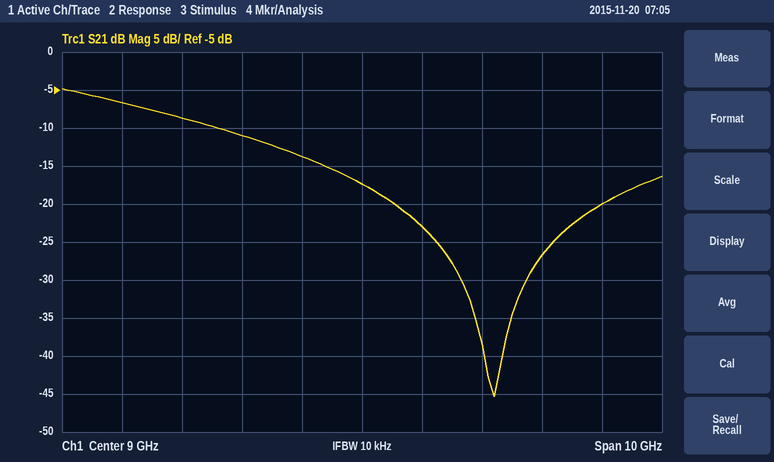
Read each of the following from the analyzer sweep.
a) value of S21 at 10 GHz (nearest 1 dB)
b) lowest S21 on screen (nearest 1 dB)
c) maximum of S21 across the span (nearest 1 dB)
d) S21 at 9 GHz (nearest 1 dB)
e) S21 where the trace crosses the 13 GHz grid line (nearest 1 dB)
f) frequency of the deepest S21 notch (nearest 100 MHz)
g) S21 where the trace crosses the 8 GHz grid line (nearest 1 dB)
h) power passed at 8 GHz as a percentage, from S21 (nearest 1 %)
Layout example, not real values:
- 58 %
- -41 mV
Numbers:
- -23 dB
- -45 dB
- -5 dB
- -17 dB
- -20 dB
- 11.2 GHz
- -14 dB
- 4 %
